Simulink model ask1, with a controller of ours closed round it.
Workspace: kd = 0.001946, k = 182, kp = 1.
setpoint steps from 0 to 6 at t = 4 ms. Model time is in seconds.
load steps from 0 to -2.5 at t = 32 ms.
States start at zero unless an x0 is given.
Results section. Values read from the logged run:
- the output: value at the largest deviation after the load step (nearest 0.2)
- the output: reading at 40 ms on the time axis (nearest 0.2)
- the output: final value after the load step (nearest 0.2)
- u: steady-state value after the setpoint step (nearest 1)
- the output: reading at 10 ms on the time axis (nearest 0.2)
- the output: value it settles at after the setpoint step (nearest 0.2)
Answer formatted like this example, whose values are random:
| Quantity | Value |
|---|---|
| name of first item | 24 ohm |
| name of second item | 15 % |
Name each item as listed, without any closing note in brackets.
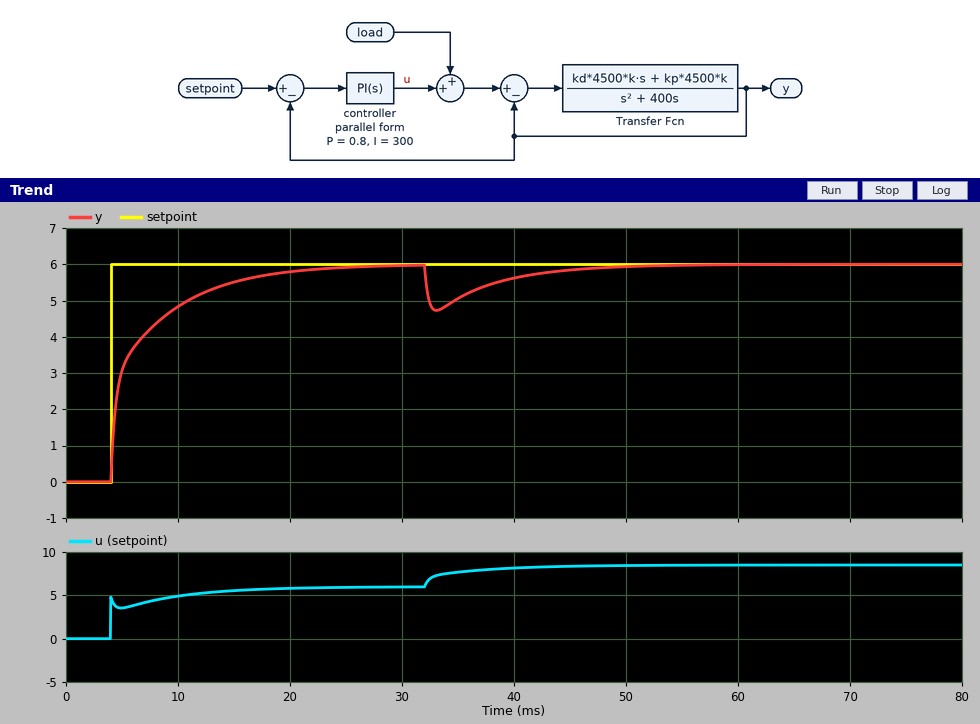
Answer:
| Quantity | Value |
|---|---|
| the output: value at the largest deviation after the load step | 4.8 |
| the output: reading at 40 ms on the time axis | 5.6 |
| the output: final value after the load step | 6.0 |
| u: steady-state value after the setpoint step | 6 |
| the output: reading at 10 ms on the time axis | 4.8 |
| the output: value it settles at after the setpoint step | 6.0 |
